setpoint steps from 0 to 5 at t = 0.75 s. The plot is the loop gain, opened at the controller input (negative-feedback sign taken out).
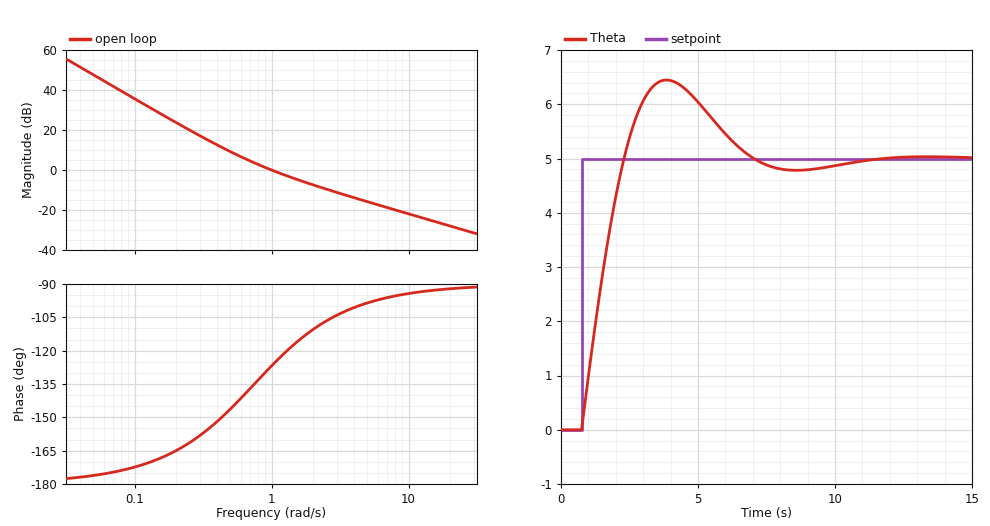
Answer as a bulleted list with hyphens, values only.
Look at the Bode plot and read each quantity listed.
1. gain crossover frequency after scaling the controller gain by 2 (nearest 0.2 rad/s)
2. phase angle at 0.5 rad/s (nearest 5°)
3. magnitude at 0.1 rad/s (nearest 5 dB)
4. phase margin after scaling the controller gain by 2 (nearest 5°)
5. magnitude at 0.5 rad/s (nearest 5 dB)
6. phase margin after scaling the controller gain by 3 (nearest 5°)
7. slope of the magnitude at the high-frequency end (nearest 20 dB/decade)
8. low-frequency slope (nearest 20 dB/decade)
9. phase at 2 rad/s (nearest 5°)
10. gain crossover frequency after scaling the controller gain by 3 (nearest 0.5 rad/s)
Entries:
- 1.8 rad/s
- -145°
- 35 dB
- 65°
- 10 dB
- 75°
- -20 dB/decade
- -40 dB/decade
- -110°
- 2.5 rad/s
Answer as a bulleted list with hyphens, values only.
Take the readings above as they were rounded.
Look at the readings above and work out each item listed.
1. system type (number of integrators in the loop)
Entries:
- 2
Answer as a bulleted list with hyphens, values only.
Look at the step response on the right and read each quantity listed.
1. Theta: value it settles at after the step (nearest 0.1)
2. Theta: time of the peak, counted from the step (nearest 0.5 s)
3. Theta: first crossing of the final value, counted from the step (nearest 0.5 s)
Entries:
- 5.0
- 3.0 s
- 1.5 s
